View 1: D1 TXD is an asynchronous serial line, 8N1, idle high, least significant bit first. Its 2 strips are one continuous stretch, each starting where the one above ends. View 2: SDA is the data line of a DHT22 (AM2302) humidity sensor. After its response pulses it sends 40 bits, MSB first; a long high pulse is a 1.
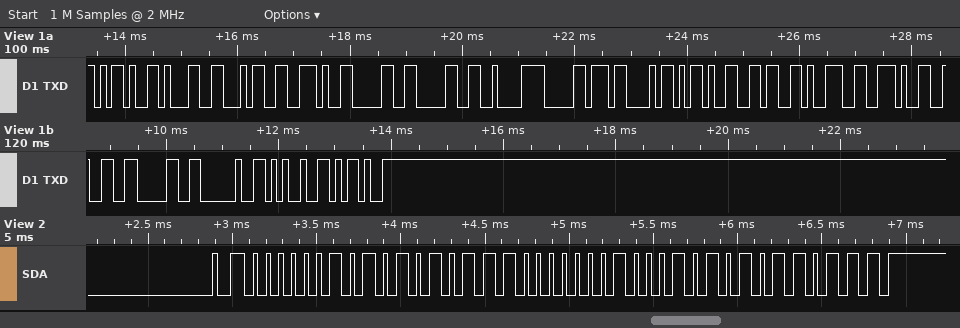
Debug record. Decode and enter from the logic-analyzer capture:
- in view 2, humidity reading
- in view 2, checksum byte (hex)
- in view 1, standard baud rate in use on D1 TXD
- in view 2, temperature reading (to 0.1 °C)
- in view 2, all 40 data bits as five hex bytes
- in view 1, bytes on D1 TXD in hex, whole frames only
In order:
68.3 %
0xB7
9600 baud
-13.8 °C
02 AB 80 8A B7
2D 31 34 2E 30 30 C2 B0 43 2D 36 39 2E 32 30 20 25 2D
